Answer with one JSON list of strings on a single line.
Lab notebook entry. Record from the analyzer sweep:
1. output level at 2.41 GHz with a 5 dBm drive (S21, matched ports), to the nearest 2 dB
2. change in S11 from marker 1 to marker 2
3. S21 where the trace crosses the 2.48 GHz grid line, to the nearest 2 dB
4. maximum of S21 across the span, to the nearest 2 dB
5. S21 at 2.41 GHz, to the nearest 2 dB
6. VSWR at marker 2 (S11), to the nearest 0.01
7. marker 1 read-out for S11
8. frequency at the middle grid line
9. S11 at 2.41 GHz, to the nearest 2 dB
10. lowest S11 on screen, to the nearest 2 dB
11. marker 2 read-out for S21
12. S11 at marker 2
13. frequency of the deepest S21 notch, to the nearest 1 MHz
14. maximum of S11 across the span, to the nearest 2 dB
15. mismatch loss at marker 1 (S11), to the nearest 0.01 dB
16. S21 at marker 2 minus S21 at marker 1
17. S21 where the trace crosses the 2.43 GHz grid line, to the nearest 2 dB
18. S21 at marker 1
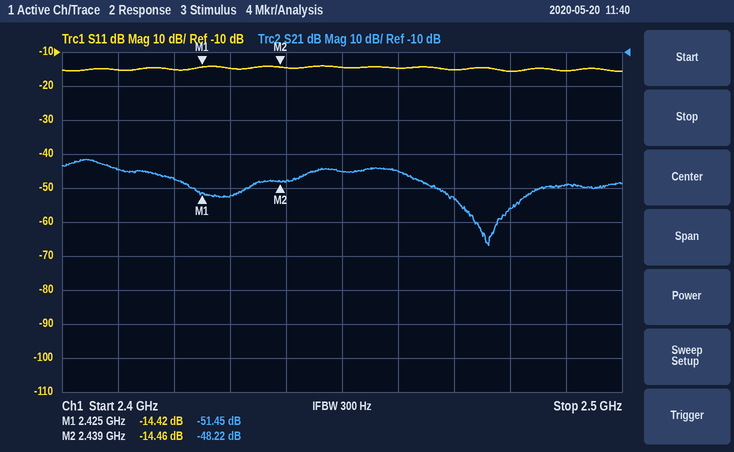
["-40 dBm", "-0.04 dB", "-56 dB", "-42 dB", "-44 dB", "1.47", "-14.42 dB", "2.45 GHz", "-16 dB", "-16 dB", "-48.22 dB", "-14.46 dB", "2.476 GHz", "-14 dB", "0.16 dB", "3.23 dB", "-52 dB", "-51.45 dB"]
